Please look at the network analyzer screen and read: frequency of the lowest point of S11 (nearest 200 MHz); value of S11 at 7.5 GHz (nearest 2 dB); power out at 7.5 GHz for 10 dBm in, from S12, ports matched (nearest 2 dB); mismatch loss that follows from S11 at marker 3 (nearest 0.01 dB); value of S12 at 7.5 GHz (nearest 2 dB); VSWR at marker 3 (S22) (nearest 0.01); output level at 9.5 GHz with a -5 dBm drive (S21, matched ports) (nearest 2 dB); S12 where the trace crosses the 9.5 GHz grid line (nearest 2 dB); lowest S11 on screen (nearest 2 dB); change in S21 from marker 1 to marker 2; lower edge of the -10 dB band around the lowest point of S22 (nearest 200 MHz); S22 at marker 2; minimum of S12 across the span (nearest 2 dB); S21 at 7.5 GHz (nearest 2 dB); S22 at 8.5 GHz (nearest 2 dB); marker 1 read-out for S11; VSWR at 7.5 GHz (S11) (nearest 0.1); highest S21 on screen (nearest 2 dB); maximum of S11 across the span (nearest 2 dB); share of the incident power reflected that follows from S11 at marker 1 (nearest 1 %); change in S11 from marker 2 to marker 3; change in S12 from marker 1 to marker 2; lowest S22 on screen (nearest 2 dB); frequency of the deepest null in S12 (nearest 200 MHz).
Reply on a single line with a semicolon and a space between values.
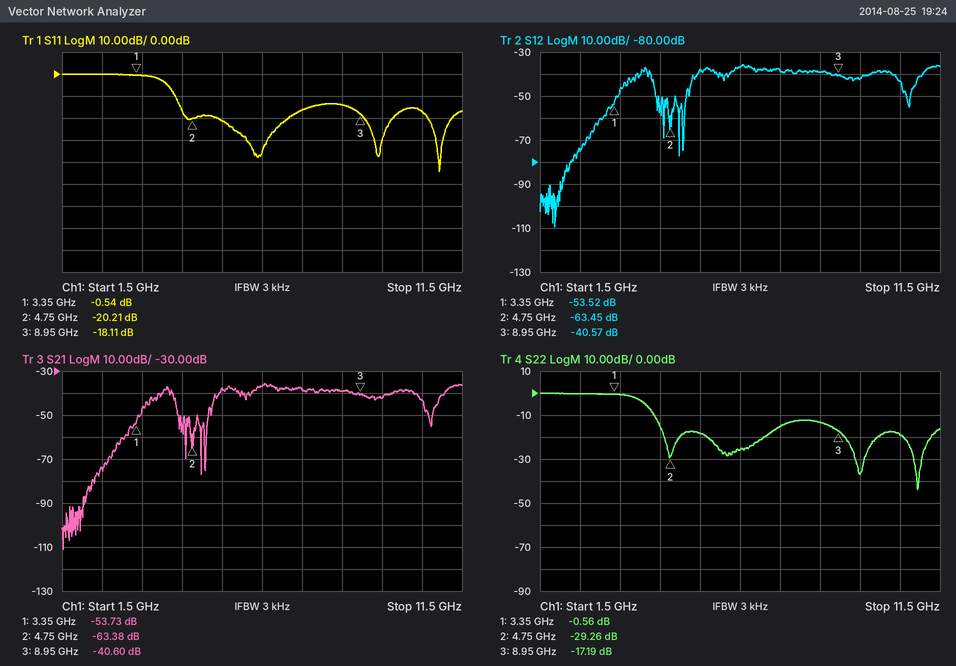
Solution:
11.0 GHz; -16 dB; -28 dBm; 0.07 dB; -38 dB; 1.32; -48 dBm; -42 dB; -44 dB; -9.65 dB; 4.4 GHz; -29.26 dB; -110 dB; -38 dB; -14 dB; -0.54 dB; 1.4; -36 dB; 0 dB; 88 %; 2.10 dB; -9.93 dB; -44 dB; 1.8 GHz
